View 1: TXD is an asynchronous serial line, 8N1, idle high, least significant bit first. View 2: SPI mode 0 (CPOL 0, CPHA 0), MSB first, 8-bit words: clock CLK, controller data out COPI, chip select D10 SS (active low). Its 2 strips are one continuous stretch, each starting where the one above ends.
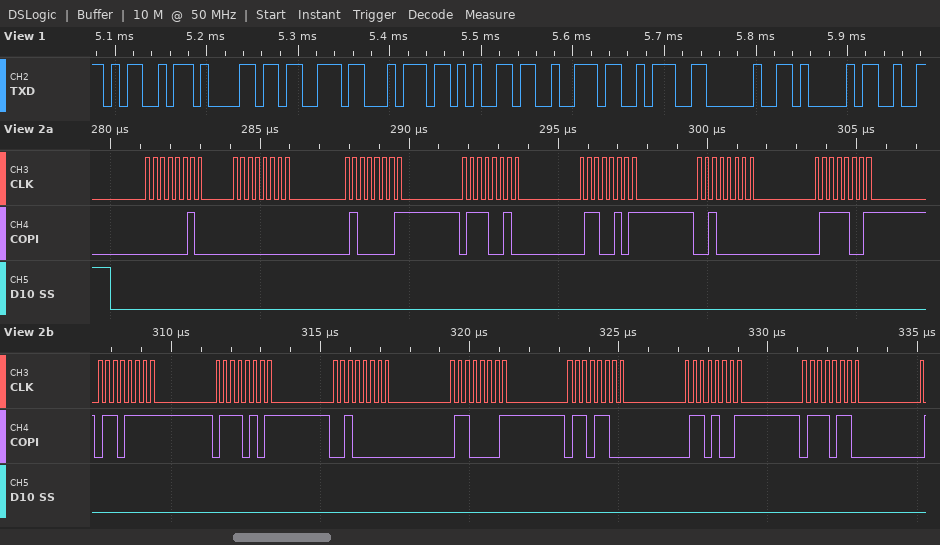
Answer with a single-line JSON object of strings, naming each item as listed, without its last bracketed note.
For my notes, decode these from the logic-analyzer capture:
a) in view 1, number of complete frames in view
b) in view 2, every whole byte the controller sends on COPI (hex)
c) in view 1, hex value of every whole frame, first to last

{"in view 1, number of complete frames in view": "9", "in view 2, every whole byte the controller sends on COPI": "02 00 41 72 65 20 79 6F 75 20 61 6C 69 76", "in view 1, hex value of every whole frame, first to last": "0x4D 0x61 0x73 0x74 0x65 0x72 0x3A 0x20 0x41"}
